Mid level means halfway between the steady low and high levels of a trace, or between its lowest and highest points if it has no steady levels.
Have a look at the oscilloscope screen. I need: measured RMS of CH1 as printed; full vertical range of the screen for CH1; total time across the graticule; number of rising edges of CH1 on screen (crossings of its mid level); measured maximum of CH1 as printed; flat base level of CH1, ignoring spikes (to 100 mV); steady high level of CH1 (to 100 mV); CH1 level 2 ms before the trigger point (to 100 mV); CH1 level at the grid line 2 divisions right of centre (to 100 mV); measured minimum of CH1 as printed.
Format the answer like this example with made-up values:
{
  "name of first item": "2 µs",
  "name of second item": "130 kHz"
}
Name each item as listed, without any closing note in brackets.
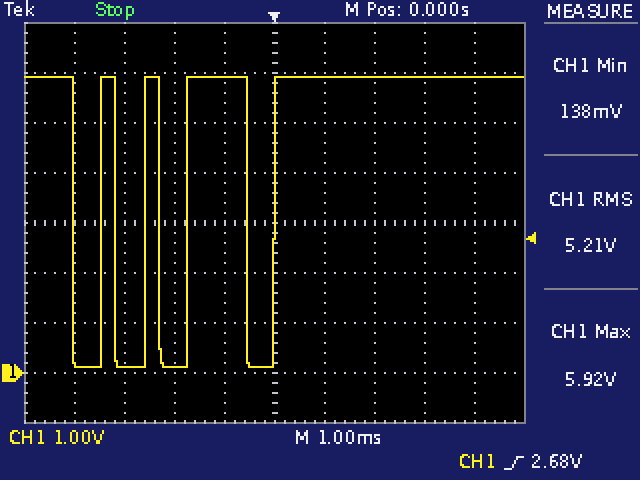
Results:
{
  "measured RMS of CH1 as printed": "5.21 V",
  "full vertical range of the screen for CH1": "8 V",
  "total time across the graticule": "10 ms",
  "number of rising edges of CH1 on screen": "4",
  "measured maximum of CH1 as printed": "5.92 V",
  "flat base level of CH1, ignoring spikes": "100 mV",
  "steady high level of CH1": "5.9 V",
  "CH1 level 2 ms before the trigger point": "100 mV",
  "CH1 level at the grid line 2 divisions right of centre": "5.9 V",
  "measured minimum of CH1 as printed": "138 mV"
}
